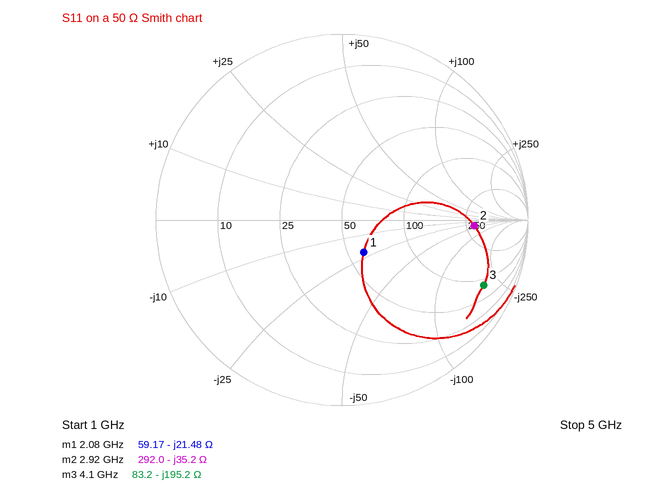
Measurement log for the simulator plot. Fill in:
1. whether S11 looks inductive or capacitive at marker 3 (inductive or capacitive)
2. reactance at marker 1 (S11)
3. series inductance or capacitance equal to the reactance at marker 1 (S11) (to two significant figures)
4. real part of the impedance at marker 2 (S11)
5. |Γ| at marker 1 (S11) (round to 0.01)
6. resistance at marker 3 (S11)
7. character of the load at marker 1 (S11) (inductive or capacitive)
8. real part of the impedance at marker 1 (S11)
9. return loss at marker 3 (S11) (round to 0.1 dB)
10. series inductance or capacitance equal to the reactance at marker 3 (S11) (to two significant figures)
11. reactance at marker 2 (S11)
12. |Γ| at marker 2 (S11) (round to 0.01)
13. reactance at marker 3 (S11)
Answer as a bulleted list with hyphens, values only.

- capacitive
- -21.48 Ω
- 3.6 pF
- 292.0 Ω
- 0.21
- 83.2 Ω
- capacitive
- 59.17 Ω
- 1.5 dB
- 200 fF
- -35.2 Ω
- 0.71
- -195.2 Ω
